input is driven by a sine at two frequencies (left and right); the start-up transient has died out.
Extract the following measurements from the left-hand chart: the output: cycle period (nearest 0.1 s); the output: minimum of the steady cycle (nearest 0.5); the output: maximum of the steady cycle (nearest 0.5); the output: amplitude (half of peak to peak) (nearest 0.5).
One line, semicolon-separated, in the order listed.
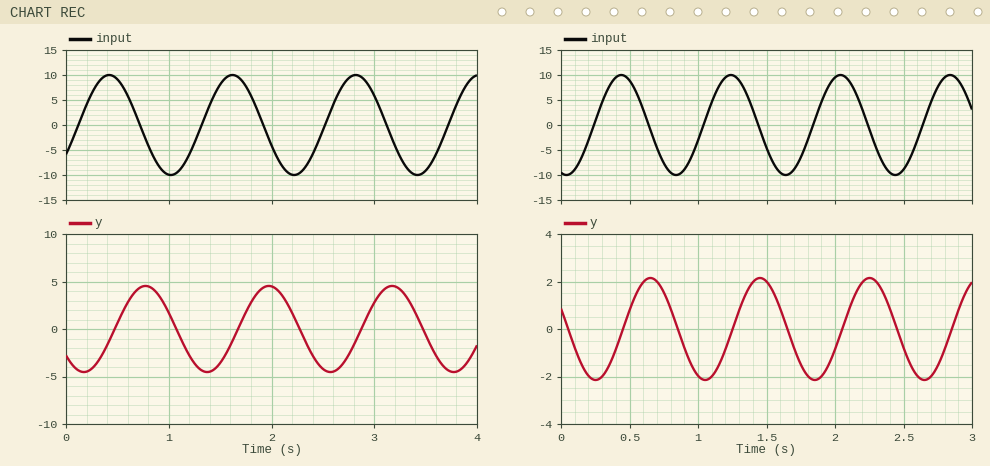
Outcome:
1.2 s; -4.5; 4.5; 4.5
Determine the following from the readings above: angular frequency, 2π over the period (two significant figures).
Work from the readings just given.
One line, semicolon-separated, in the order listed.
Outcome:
5.2 rad/s
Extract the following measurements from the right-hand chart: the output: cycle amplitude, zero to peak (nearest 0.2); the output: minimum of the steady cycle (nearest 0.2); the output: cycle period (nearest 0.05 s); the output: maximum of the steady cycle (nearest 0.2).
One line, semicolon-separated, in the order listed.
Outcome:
2.2; -2.2; 0.80 s; 2.2
